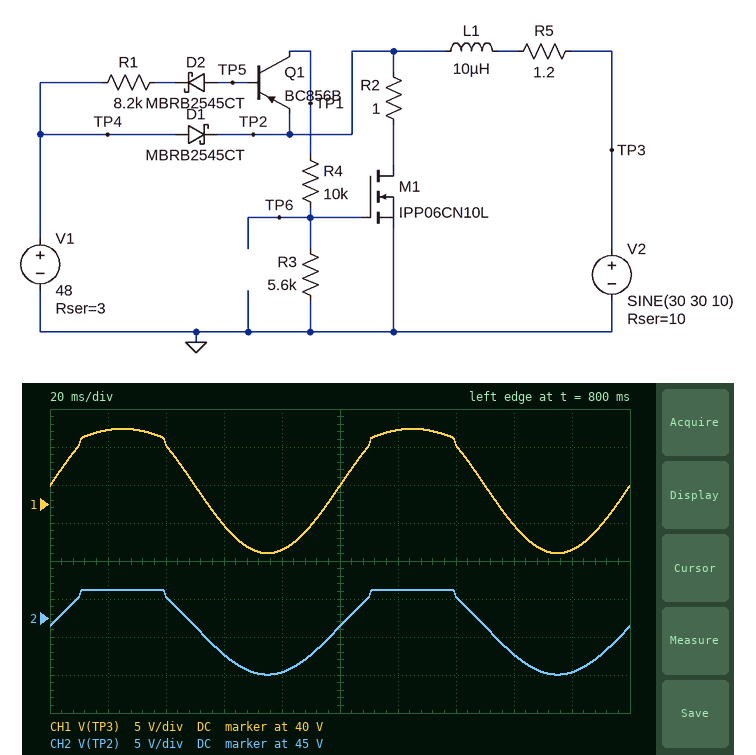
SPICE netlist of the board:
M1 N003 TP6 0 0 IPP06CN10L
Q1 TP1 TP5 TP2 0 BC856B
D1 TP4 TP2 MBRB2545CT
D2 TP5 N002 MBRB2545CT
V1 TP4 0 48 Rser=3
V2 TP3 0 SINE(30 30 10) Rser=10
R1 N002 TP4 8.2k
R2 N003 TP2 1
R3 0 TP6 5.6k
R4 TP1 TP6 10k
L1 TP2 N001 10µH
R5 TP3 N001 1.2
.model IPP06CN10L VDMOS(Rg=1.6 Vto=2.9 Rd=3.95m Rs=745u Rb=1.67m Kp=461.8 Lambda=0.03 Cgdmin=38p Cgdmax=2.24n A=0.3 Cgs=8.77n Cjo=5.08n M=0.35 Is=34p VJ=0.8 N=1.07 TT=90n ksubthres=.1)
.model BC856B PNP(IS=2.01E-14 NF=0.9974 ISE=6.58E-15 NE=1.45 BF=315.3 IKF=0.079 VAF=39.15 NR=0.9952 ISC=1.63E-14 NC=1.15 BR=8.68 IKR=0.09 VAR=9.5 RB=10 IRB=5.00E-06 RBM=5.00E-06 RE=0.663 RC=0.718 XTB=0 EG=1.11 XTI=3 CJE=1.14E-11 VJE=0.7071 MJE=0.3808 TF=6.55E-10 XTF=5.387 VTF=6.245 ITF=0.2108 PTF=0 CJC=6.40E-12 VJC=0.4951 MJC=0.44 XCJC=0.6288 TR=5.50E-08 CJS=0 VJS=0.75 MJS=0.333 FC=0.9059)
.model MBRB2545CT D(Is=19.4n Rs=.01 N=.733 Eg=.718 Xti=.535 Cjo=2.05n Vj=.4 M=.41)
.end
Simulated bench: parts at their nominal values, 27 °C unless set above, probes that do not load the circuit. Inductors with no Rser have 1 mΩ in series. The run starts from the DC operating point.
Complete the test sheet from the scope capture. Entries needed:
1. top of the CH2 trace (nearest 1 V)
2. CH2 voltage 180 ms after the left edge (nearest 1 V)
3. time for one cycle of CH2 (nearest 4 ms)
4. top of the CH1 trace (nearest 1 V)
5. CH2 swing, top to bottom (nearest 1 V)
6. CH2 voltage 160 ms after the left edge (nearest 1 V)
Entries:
49 V
38 V
100 ms
50 V
11 V
40 V
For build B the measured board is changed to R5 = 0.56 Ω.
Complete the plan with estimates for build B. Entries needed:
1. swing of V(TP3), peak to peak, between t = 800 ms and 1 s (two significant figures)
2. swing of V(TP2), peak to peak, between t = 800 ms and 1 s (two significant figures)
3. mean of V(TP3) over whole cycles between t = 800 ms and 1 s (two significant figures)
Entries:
14 V
12 V
43 V
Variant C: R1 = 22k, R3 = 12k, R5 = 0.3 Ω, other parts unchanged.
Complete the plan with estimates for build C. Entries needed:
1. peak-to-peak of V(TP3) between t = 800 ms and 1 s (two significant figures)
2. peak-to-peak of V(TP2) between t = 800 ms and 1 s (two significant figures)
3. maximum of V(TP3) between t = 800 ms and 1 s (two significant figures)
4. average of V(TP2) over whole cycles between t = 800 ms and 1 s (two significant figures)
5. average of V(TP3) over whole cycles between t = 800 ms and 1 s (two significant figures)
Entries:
13 V
12 V
49 V
43 V
43 V
